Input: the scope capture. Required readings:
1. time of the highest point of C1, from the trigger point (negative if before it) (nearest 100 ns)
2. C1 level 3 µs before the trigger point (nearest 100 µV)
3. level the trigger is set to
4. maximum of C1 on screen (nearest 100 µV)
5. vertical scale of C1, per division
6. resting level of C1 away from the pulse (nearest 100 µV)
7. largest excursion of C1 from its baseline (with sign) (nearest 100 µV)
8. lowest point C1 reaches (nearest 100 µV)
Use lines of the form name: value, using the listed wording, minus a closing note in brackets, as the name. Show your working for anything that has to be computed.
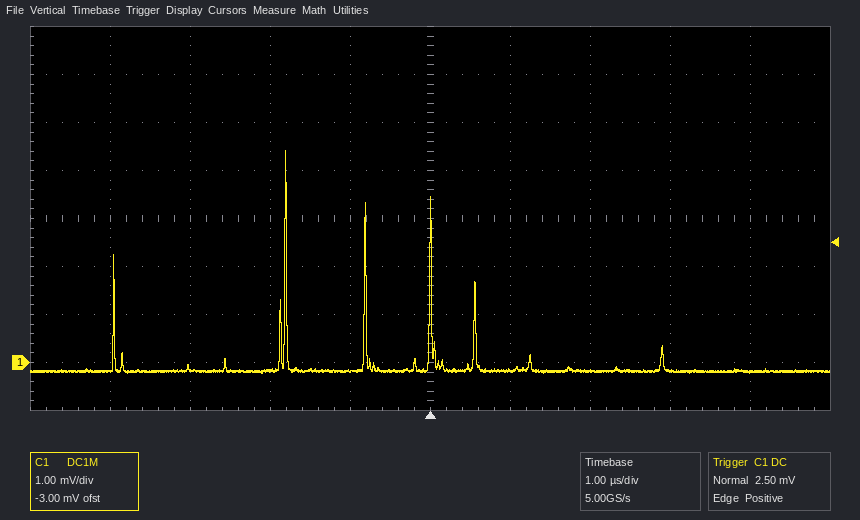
time of the highest point of C1, from the trigger point (negative if before it): -1.8 µs
C1 level 3 µs before the trigger point: -100 µV
level the trigger is set to: 2.50 mV
maximum of C1 on screen: 4.4 mV
vertical scale of C1, per division: 1 mV
resting level of C1 away from the pulse: -200 µV
largest excursion of C1 from its baseline (with sign): 4.4 mV − (-200 µV) = +4.6 mV
lowest point C1 reaches: -200 µV
